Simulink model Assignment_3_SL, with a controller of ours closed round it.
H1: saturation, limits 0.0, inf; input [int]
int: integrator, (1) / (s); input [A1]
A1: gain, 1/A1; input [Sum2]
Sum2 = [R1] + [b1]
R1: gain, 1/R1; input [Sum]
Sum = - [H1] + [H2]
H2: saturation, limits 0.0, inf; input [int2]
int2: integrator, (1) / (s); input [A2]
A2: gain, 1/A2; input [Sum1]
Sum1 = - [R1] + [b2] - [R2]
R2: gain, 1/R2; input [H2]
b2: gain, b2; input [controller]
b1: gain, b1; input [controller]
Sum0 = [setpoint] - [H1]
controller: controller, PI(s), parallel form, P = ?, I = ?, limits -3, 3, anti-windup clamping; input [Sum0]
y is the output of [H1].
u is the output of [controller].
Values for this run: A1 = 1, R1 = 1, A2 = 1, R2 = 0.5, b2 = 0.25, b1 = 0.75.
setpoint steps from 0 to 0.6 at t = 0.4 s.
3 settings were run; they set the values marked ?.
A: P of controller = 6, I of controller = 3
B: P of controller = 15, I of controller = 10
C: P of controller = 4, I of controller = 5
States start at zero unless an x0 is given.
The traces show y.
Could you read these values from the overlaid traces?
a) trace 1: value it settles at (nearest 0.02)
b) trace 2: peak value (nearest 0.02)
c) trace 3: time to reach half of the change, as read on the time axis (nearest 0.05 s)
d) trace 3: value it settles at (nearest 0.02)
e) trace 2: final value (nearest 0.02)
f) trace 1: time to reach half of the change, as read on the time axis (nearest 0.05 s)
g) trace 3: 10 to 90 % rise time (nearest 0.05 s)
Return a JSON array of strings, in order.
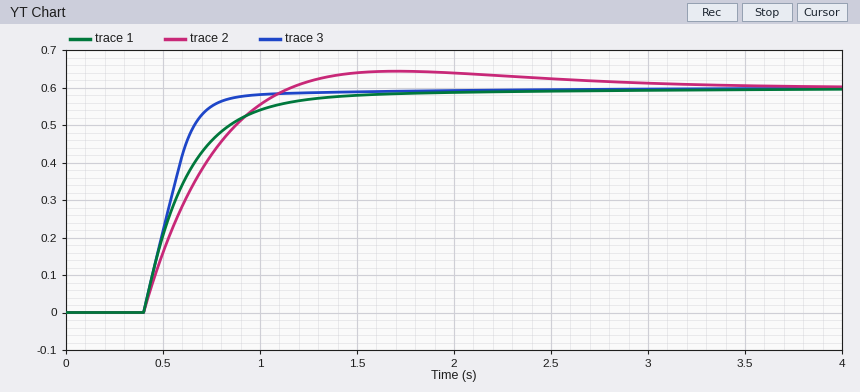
["0.60", "0.64", "0.55 s", "0.60", "0.60", "0.55 s", "0.30 s"]
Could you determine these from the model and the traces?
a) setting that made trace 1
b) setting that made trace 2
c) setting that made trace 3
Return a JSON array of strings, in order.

["A", "C", "B"]
